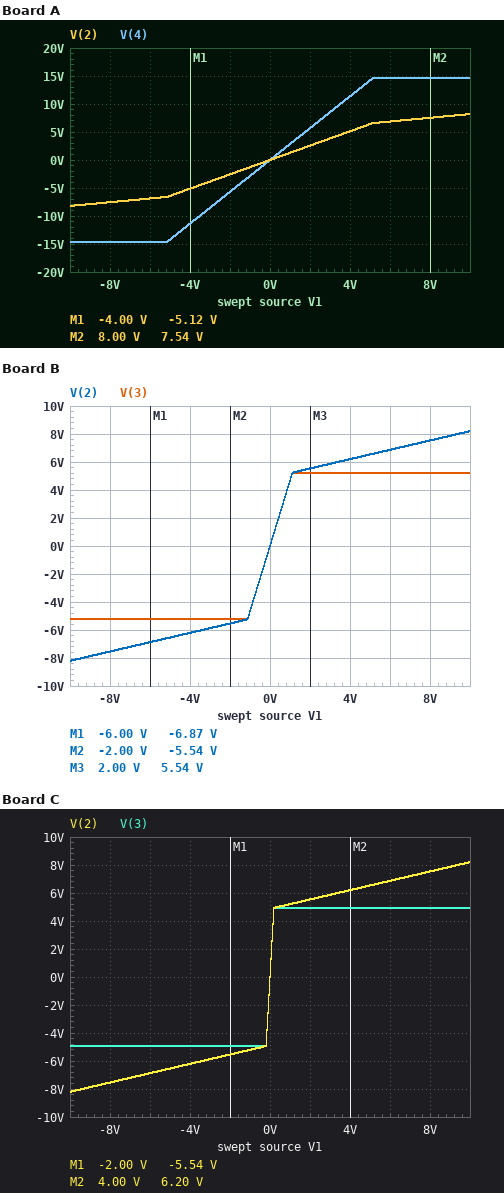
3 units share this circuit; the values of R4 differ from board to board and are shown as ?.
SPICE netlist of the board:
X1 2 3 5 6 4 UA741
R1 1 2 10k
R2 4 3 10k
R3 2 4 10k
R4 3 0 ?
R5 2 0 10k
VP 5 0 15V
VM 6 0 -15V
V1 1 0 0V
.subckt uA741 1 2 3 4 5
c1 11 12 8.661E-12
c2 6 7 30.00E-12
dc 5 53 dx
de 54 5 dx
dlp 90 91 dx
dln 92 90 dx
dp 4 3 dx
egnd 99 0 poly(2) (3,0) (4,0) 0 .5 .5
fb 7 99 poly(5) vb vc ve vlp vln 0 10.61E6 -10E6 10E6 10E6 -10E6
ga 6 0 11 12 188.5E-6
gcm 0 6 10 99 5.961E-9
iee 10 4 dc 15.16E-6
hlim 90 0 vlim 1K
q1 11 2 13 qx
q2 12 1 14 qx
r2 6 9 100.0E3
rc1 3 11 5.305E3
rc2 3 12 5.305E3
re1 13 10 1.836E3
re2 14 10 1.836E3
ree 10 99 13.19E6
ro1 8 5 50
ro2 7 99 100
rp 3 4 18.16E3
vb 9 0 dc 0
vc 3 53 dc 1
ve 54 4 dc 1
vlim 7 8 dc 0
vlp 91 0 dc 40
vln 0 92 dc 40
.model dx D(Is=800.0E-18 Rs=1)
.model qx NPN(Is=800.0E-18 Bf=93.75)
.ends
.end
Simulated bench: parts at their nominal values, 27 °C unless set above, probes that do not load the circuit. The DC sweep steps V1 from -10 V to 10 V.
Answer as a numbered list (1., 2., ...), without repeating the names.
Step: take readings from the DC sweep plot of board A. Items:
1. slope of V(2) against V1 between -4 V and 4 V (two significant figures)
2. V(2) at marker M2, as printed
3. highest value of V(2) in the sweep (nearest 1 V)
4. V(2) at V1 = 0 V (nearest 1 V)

1. 1.3 V/V
2. 7.54 V
3. 8 V
4. 0 V
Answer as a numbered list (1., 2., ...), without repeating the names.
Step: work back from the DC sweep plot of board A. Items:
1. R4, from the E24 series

1. 8.2 kΩ
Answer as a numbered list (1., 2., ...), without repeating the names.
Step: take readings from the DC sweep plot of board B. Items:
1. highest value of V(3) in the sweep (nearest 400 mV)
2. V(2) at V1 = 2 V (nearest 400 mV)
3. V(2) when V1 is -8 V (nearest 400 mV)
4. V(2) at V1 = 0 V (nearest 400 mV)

1. 5.2 V
2. 5.6 V
3. -7.6 V
4. 0 V
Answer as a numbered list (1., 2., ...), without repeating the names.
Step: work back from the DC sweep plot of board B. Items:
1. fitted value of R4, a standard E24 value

1. 5.6 kΩ
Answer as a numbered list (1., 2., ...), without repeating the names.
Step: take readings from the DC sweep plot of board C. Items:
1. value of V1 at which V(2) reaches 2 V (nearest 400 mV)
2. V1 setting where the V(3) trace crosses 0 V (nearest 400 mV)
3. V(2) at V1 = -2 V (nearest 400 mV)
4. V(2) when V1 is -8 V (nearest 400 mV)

1. 0 V
2. 0 V
3. -5.6 V
4. -7.6 V
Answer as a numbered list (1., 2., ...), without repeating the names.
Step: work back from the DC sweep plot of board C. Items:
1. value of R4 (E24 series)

1. 5.1 kΩ
